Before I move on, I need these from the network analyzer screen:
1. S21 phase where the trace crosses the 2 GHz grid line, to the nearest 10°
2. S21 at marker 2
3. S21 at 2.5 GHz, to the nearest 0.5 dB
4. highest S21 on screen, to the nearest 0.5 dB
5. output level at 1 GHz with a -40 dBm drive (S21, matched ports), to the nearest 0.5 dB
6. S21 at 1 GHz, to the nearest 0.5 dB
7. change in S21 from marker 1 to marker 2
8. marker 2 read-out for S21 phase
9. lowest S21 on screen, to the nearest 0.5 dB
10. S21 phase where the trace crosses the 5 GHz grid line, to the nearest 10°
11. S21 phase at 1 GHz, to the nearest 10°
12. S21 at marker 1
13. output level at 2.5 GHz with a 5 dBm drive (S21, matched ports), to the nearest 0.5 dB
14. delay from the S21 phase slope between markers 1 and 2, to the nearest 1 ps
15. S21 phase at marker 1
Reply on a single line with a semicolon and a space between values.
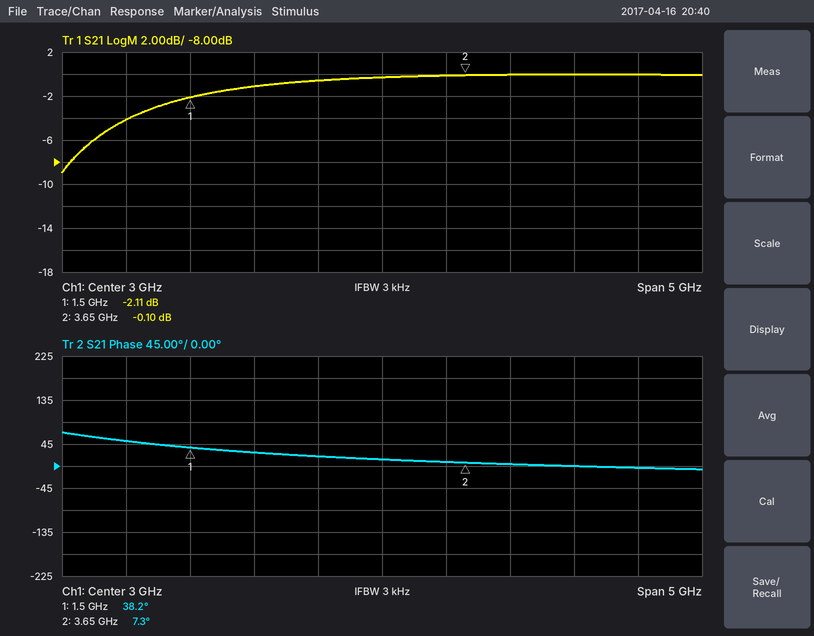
30°; -0.10 dB; -0.5 dB; 0.0 dB; -44.0 dBm; -4.0 dB; 2.01 dB; 7.3°; -9.0 dB; 0°; 50°; -2.11 dB; 4.5 dBm; 40 ps; 38.2°
